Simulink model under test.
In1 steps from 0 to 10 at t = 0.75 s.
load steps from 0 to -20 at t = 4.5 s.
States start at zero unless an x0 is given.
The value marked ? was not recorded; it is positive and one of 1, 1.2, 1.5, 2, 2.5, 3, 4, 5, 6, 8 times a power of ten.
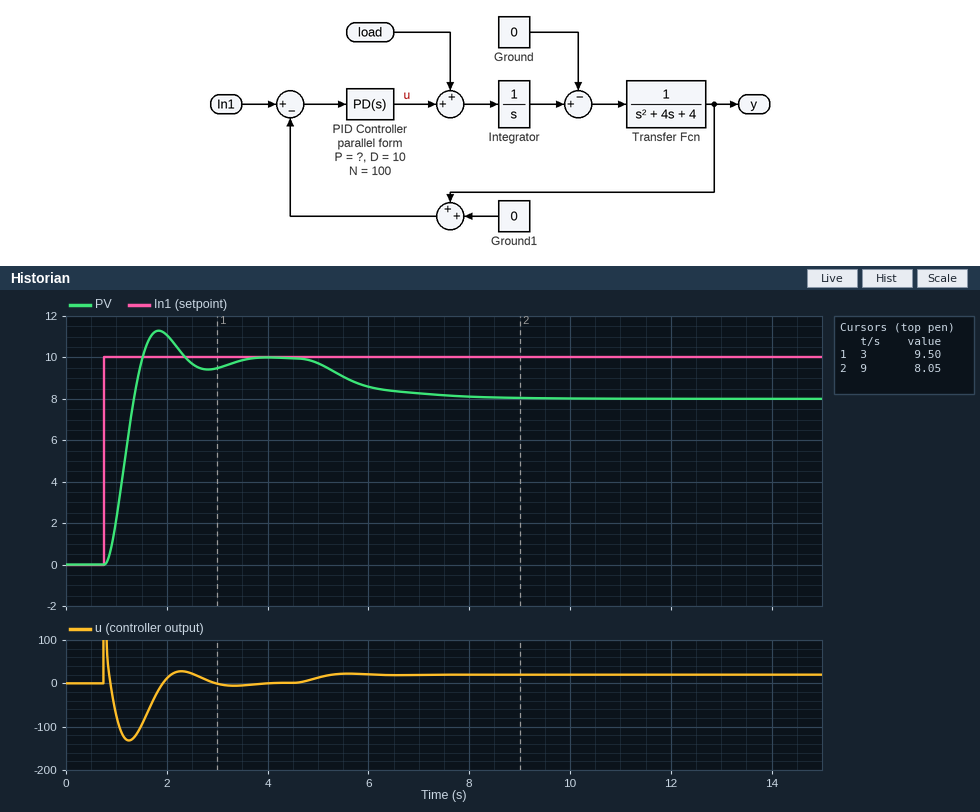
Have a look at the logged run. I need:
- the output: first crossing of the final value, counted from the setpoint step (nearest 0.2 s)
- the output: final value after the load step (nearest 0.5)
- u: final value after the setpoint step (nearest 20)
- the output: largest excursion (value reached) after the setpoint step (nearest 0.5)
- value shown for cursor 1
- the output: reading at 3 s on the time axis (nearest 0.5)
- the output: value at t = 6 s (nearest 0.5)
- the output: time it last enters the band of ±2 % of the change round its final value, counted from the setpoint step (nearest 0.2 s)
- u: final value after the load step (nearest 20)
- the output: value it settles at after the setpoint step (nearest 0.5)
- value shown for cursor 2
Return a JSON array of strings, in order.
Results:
["0.8 s", "8.0", "0", "11.5", "9.50", "9.5", "8.5", "2.6 s", "20", "10.0", "8.05"]
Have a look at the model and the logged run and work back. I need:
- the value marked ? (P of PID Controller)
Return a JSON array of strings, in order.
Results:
["10"]
